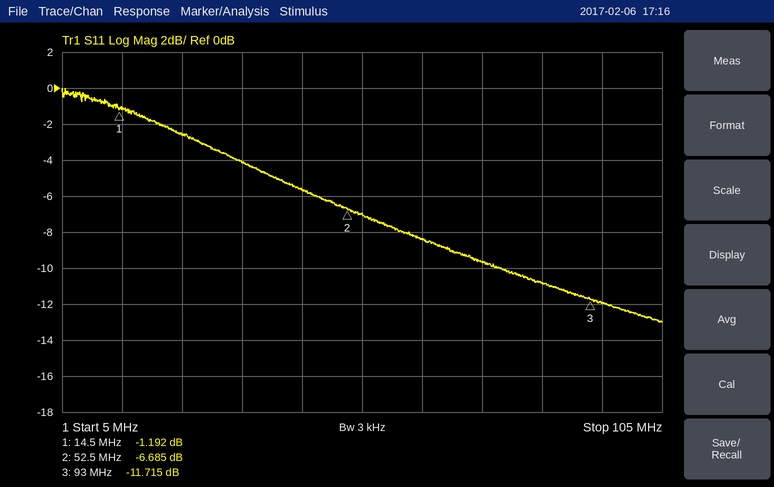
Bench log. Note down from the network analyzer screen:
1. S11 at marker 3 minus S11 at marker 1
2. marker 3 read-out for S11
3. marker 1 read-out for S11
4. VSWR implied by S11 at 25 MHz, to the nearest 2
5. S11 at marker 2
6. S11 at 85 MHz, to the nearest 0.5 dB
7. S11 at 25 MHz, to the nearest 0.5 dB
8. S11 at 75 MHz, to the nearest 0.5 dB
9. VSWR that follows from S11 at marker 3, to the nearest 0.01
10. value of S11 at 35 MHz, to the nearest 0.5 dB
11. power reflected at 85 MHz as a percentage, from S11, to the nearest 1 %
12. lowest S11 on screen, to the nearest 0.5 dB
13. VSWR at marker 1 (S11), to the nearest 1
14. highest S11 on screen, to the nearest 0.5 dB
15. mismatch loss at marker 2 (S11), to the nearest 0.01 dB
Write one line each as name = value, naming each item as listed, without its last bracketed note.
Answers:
S11 at marker 3 minus S11 at marker 1 = -10.523 dB
marker 3 read-out for S11 = -11.715 dB
marker 1 read-out for S11 = -1.192 dB
VSWR implied by S11 at 25 MHz, to the nearest 2 = 6
S11 at marker 2 = -6.685 dB
S11 at 85 MHz, to the nearest 0.5 dB = -11.0 dB
S11 at 25 MHz, to the nearest 0.5 dB = -2.5 dB
S11 at 75 MHz, to the nearest 0.5 dB = -9.5 dB
VSWR that follows from S11 at marker 3, to the nearest 0.01 = 1.70
value of S11 at 35 MHz, to the nearest 0.5 dB = -4.0 dB
power reflected at 85 MHz as a percentage, from S11, to the nearest 1 % = 8 %
lowest S11 on screen, to the nearest 0.5 dB = -13.0 dB
VSWR at marker 1 (S11), to the nearest 1 = 15
highest S11 on screen, to the nearest 0.5 dB = 0.0 dB
mismatch loss at marker 2 (S11), to the nearest 0.01 dB = 1.05 dB
